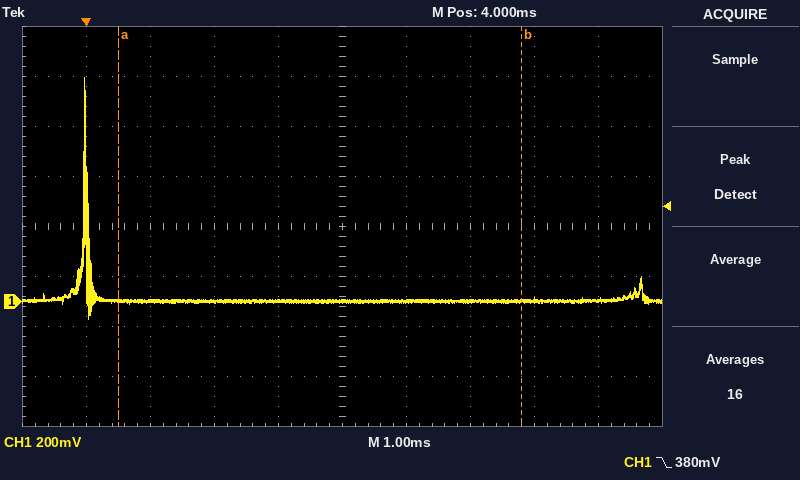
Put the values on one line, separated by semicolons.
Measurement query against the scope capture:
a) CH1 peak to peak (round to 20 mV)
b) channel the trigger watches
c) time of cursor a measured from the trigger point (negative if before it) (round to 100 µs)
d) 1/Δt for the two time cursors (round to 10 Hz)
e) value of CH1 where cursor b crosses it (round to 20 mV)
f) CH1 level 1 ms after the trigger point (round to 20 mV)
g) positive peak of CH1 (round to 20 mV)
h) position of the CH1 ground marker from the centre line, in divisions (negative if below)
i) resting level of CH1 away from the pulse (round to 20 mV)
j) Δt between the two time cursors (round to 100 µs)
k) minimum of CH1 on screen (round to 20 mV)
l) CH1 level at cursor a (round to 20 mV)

960 mV; CH1; +500 µs; 160 Hz; 0 mV; 0 mV; 900 mV; -1.5 div; 0 mV; 6.3 ms; -60 mV; 0 mV
